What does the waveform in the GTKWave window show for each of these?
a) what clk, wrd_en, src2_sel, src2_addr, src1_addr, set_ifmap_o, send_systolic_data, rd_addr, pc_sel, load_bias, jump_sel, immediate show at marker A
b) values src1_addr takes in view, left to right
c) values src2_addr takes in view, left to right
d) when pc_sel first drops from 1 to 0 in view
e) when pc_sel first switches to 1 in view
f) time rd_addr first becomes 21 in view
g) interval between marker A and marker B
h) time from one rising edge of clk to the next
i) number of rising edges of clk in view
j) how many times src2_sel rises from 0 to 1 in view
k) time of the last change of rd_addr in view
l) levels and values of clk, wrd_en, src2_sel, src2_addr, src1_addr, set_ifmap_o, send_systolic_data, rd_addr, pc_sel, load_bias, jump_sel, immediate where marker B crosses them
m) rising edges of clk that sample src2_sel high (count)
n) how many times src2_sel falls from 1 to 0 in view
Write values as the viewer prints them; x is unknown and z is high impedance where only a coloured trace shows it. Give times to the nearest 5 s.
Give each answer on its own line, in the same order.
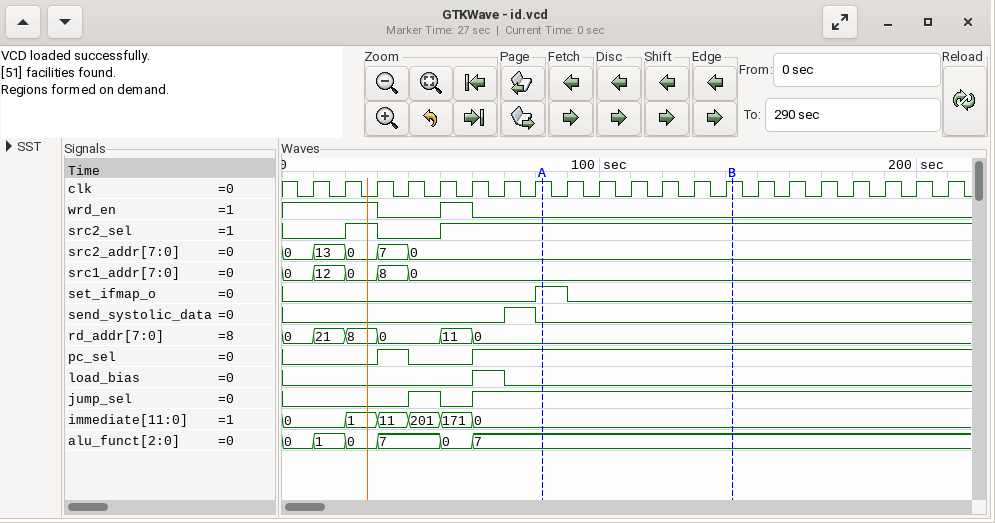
clk=1, wrd_en=0, src2_sel=1, src2_addr=0, src1_addr=0, set_ifmap_o=1, send_systolic_data=0, rd_addr=0, pc_sel=1, load_bias=0, jump_sel=1, immediate=0
0, 12, 0, 8, 0
0, 13, 0, 7, 0
40 s
30 s
10 s
60 s
10 s
21
2
60 s
clk=1, wrd_en=0, src2_sel=1, src2_addr=0, src1_addr=0, set_ifmap_o=0, send_systolic_data=0, rd_addr=0, pc_sel=1, load_bias=0, jump_sel=1, immediate=0
17
1
